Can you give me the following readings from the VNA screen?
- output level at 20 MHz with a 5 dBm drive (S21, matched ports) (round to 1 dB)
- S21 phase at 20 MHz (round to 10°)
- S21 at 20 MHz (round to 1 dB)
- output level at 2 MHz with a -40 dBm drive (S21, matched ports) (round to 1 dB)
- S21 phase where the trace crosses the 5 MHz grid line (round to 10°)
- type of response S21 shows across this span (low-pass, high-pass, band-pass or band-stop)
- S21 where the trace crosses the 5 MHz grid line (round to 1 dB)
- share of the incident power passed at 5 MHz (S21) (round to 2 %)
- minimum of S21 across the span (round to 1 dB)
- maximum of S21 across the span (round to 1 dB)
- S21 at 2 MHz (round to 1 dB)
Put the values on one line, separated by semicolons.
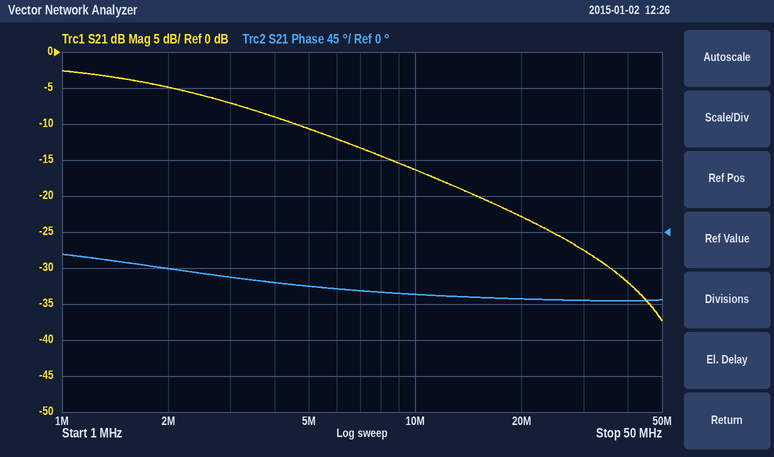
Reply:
-18 dBm; -80°; -23 dB; -45 dBm; -70°; low-pass; -11 dB; 8 %; -37 dB; -3 dB; -5 dB
